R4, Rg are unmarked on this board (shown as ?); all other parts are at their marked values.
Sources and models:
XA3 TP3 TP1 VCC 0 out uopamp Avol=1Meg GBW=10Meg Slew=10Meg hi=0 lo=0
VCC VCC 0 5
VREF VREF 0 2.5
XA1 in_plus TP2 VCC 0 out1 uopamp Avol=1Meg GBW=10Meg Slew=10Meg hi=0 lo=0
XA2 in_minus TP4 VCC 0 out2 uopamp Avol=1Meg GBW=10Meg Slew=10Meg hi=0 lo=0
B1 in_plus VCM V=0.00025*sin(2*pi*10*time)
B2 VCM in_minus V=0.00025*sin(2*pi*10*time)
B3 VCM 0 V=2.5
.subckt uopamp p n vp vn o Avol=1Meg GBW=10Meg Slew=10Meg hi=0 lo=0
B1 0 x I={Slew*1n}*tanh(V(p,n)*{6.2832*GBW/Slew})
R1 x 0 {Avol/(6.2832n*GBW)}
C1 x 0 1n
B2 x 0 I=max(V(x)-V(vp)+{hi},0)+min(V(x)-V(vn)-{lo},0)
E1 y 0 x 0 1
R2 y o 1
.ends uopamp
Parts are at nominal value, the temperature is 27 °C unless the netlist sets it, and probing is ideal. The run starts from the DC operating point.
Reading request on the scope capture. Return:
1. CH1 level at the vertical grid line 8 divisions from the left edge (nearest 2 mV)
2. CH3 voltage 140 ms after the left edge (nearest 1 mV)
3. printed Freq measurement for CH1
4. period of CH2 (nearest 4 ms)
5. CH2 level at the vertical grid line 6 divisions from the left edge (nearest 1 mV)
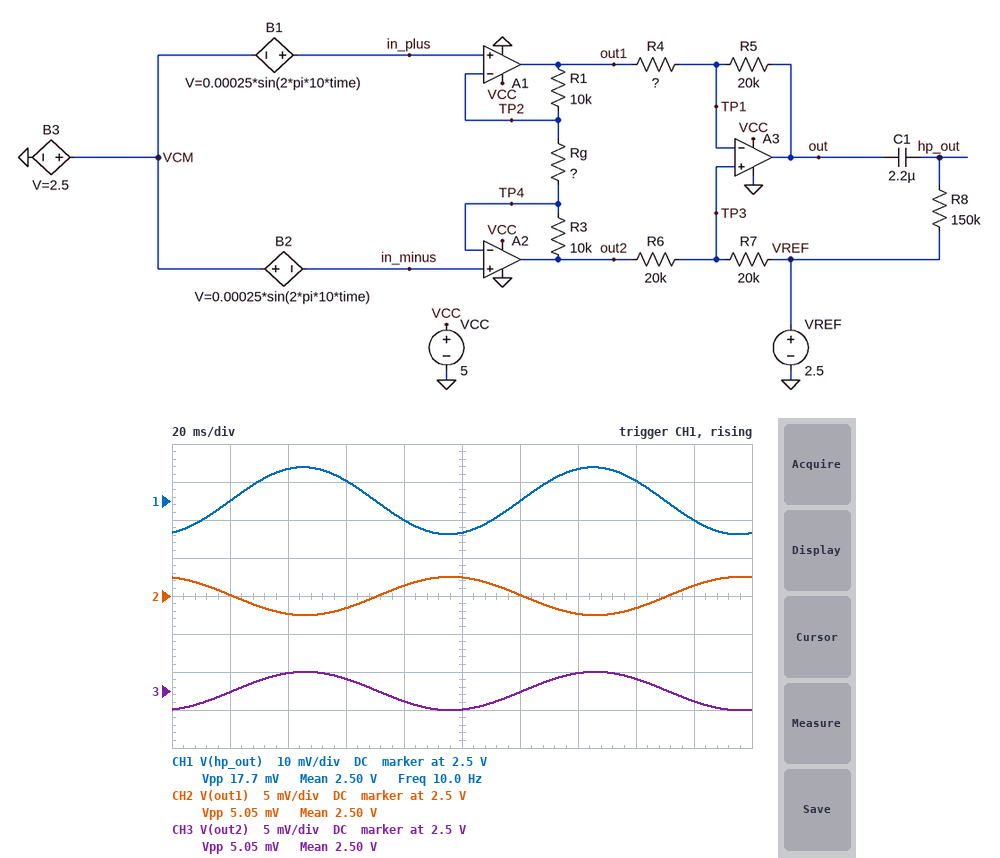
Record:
2.506 V
2.502 V
10.0 Hz
100 ms
2.500 V
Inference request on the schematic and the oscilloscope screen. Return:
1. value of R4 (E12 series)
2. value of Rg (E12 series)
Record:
10 kΩ
2.2 kΩ
